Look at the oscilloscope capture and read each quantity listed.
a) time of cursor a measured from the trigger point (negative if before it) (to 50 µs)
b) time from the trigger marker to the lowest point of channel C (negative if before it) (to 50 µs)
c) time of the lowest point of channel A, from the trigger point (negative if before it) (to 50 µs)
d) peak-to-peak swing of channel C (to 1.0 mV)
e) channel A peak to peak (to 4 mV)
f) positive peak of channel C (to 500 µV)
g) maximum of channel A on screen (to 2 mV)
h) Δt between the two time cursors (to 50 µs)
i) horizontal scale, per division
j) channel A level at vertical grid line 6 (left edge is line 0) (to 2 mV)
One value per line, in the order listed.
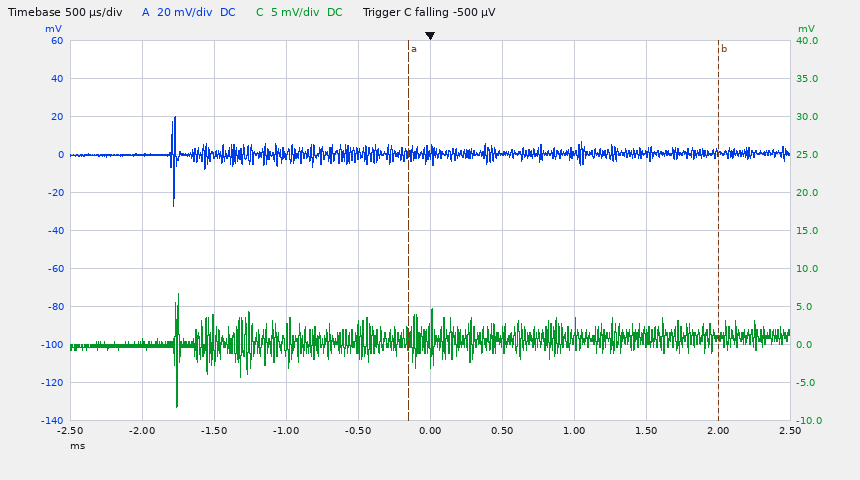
-150 µs
-1.75 ms
-1.80 ms
15.0 mV
48 mV
6.5 mV
20 mV
2.15 ms
500 µs
0 mV
